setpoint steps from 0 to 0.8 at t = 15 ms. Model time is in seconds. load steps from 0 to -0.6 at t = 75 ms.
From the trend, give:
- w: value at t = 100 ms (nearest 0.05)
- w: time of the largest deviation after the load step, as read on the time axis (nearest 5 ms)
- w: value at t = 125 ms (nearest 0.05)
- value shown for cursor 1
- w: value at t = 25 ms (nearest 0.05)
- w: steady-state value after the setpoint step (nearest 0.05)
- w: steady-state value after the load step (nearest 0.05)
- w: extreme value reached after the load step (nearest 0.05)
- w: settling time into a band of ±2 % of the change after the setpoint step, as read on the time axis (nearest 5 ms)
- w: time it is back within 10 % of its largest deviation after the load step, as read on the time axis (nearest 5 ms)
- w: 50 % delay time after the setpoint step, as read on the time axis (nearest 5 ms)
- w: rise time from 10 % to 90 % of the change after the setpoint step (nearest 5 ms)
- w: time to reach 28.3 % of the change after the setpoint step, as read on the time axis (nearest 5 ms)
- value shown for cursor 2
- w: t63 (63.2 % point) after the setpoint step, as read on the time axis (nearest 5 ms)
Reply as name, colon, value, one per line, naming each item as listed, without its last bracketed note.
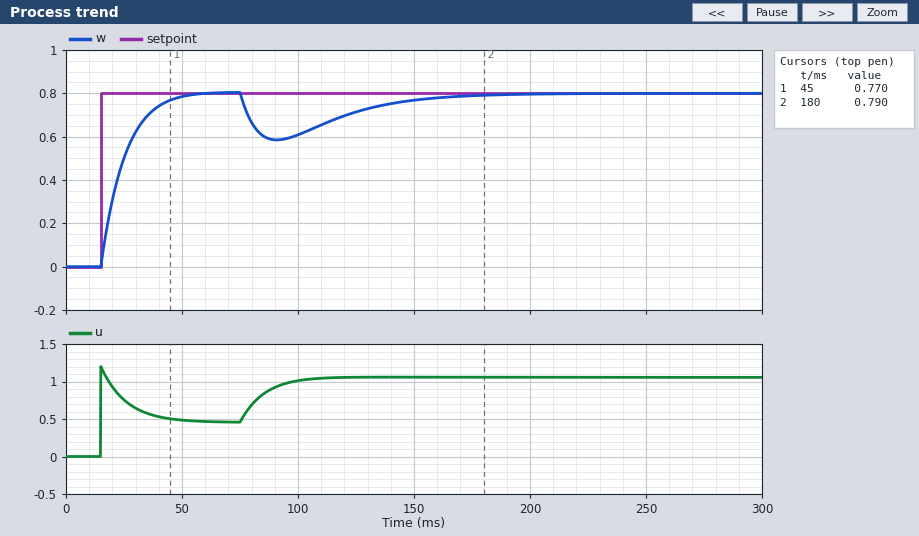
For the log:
w: value at t = 100 ms: 0.60
w: time of the largest deviation after the load step, as read on the time axis: 90 ms
w: value at t = 125 ms: 0.70
value shown for cursor 1: 0.770
w: value at t = 25 ms: 0.50
w: steady-state value after the setpoint step: 0.80
w: steady-state value after the load step: 0.80
w: extreme value reached after the load step: 0.60
w: settling time into a band of ±2 % of the change after the setpoint step, as read on the time axis: 50 ms
w: time it is back within 10 % of its largest deviation after the load step, as read on the time axis: 160 ms
w: 50 % delay time after the setpoint step, as read on the time axis: 20 ms
w: rise time from 10 % to 90 % of the change after the setpoint step: 20 ms
w: time to reach 28.3 % of the change after the setpoint step, as read on the time axis: 20 ms
value shown for cursor 2: 0.790
w: t63 (63.2 % point) after the setpoint step, as read on the time axis: 25 ms
